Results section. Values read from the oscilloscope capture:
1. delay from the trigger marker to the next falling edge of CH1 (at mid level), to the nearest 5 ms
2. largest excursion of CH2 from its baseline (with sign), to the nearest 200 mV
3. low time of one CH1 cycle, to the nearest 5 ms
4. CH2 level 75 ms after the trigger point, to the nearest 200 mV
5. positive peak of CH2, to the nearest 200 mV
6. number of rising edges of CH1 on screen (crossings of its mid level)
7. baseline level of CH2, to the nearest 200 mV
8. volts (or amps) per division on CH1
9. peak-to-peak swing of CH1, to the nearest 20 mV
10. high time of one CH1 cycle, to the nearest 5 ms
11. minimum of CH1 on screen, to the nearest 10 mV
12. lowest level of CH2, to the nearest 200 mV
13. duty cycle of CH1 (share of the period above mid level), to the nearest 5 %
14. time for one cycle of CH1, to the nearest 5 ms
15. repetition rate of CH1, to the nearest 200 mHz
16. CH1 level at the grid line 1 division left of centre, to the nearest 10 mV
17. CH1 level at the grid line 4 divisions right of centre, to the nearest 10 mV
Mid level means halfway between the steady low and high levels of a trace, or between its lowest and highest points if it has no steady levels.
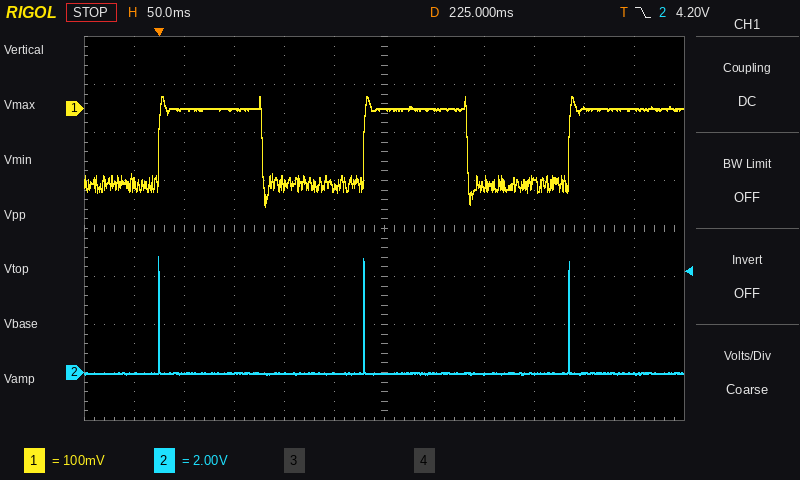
105 ms
+4.8 V
100 ms
0.0 V
4.8 V
3
0.0 V
100 mV
220 mV
105 ms
-200 mV
0.0 V
50 %
205 ms
4.8 Hz
-160 mV
0 mV
